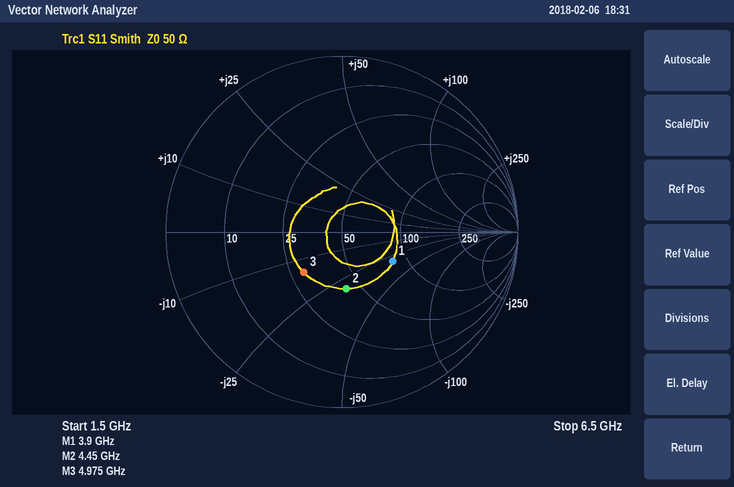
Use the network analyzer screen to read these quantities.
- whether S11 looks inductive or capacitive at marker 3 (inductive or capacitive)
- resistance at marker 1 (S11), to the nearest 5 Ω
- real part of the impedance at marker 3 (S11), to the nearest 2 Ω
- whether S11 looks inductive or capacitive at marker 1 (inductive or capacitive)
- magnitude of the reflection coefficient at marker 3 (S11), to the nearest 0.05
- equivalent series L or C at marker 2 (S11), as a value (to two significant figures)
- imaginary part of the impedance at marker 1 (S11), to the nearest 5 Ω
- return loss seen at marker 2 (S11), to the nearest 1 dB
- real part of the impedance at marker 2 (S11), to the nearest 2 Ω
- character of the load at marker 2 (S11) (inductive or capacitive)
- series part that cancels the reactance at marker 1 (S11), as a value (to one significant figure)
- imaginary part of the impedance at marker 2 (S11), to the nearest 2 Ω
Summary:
capacitive
85 Ω
30 Ω
capacitive
0.30
1.2 pF
-30 Ω
10 dB
42 Ω
capacitive
1 nH
-30 Ω
